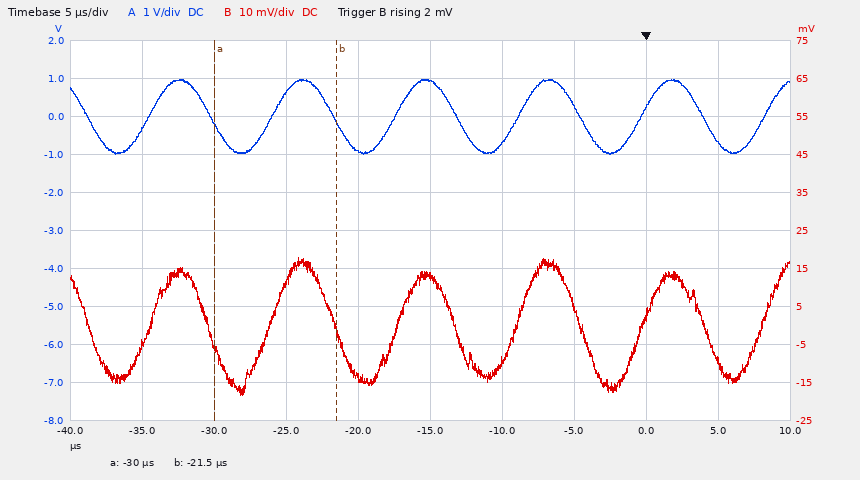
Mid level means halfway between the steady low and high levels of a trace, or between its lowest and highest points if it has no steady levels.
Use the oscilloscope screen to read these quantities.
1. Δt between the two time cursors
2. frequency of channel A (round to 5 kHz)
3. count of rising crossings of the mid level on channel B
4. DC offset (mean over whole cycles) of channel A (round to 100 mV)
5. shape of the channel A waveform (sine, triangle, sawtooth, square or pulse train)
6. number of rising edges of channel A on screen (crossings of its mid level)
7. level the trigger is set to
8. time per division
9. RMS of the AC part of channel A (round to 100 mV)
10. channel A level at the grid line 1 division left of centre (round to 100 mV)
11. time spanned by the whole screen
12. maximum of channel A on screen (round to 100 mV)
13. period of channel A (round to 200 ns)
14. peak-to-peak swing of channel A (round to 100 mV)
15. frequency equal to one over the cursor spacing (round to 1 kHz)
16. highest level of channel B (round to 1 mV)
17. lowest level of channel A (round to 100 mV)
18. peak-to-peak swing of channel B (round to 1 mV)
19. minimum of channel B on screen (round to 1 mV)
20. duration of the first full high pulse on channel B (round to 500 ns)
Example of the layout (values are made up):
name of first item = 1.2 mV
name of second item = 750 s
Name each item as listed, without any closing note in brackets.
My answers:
Δt between the two time cursors = 8.5 µs
frequency of channel A = 115 kHz
count of rising crossings of the mid level on channel B = 6
DC offset (mean over whole cycles) of channel A = 0.0 V
shape of the channel A waveform = sine
number of rising edges of channel A on screen = 6
level the trigger is set to = 2 mV
time per division = 5 µs
RMS of the AC part of channel A = 700 mV
channel A level at the grid line 1 division left of centre = -900 mV
time spanned by the whole screen = 50 µs
maximum of channel A on screen = 1.0 V
period of channel A = 8.6 µs
peak-to-peak swing of channel A = 2.0 V
frequency equal to one over the cursor spacing = 118 kHz
highest level of channel B = 18 mV
lowest level of channel A = -1.0 V
peak-to-peak swing of channel B = 36 mV
minimum of channel B on screen = -18 mV
duration of the first full high pulse on channel B = 4.0 µs
